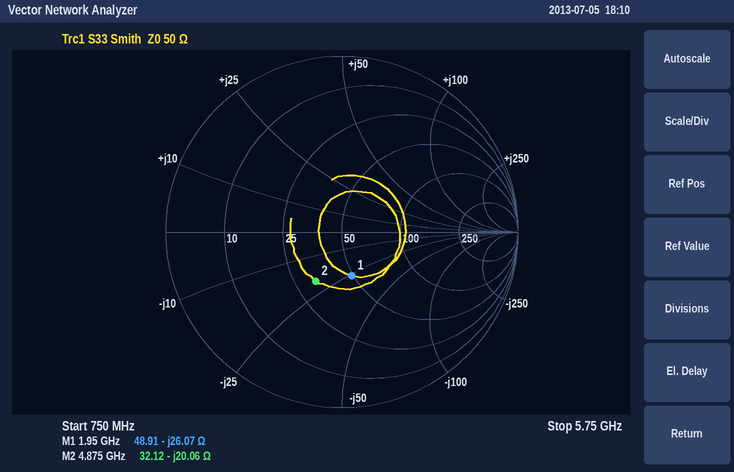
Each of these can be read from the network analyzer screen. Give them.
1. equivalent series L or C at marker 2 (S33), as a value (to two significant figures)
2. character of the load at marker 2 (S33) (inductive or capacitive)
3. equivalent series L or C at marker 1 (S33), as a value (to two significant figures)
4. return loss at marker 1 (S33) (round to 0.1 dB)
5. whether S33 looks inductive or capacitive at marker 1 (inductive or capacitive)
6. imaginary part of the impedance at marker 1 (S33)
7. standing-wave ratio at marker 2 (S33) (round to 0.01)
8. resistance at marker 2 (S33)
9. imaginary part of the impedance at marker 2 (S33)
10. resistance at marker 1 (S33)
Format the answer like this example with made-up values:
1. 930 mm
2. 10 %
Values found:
1. 1.6 pF
2. capacitive
3. 3.1 pF
4. 11.9 dB
5. capacitive
6. -26.07 Ω
7. 1.93
8. 32.12 Ω
9. -20.06 Ω
10. 48.91 Ω
